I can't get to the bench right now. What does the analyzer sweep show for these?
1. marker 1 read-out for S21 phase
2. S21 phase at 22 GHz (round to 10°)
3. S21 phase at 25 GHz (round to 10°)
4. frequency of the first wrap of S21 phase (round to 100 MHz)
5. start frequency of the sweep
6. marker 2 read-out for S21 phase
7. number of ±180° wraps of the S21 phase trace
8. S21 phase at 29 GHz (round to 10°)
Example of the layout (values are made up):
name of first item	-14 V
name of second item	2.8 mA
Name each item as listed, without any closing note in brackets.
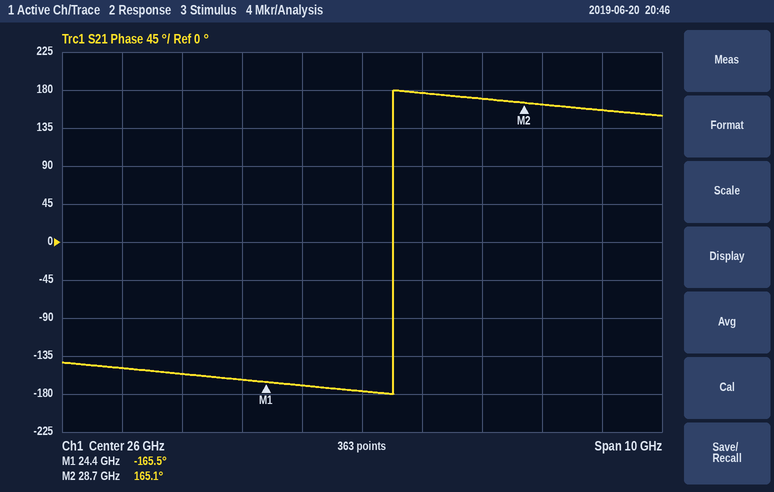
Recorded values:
marker 1 read-out for S21 phase	-165.5°
S21 phase at 22 GHz	-150°
S21 phase at 25 GHz	-170°
frequency of the first wrap of S21 phase	26.5 GHz
start frequency of the sweep	21 GHz
marker 2 read-out for S21 phase	165.1°
number of ±180° wraps of the S21 phase trace	1
S21 phase at 29 GHz	160°
